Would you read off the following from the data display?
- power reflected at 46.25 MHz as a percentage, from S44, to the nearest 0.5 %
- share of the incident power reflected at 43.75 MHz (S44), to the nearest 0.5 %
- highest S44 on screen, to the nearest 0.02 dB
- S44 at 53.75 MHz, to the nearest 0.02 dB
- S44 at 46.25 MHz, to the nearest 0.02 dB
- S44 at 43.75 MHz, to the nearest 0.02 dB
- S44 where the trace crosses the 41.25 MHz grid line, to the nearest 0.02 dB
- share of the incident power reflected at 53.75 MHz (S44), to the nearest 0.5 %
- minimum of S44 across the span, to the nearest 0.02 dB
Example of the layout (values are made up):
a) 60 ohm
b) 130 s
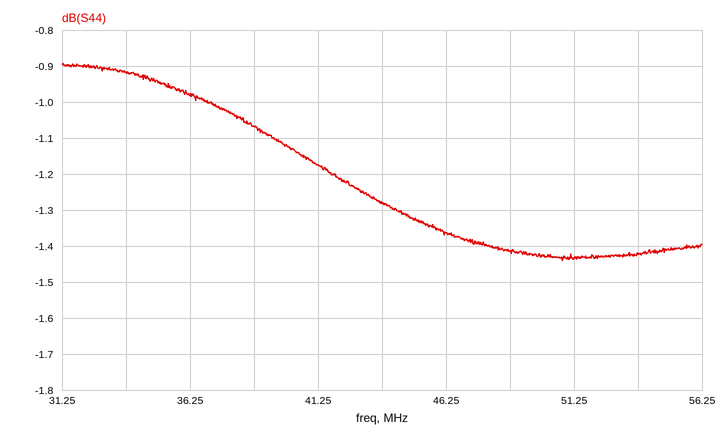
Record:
a) 73.0 %
b) 74.5 %
c) -0.90 dB
d) -1.42 dB
e) -1.36 dB
f) -1.28 dB
g) -1.18 dB
h) 72.0 %
i) -1.44 dB
